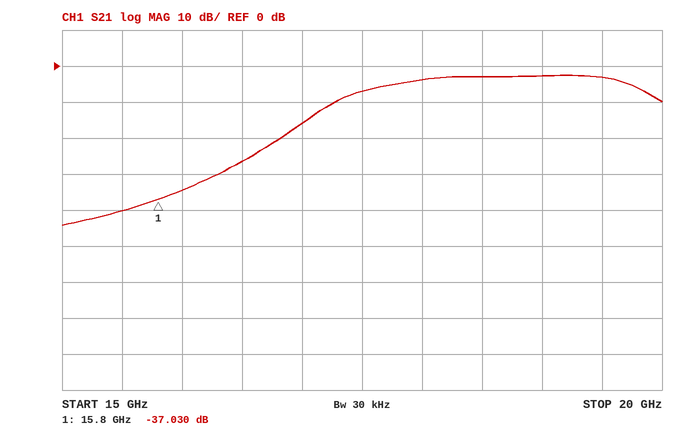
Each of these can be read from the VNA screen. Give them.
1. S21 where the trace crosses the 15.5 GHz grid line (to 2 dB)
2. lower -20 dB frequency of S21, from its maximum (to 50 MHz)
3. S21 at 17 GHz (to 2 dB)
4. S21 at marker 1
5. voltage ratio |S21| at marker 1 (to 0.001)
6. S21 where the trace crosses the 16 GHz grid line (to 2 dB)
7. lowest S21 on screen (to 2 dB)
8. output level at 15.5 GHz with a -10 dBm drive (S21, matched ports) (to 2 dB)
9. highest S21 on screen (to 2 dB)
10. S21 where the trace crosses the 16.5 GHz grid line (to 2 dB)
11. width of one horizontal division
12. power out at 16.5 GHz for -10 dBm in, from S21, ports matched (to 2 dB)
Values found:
-40 dB
16.70 GHz
-16 dB
-37.030 dB
0.014
-34 dB
-44 dB
-50 dBm
-2 dB
-26 dB
500 MHz
-36 dBm
